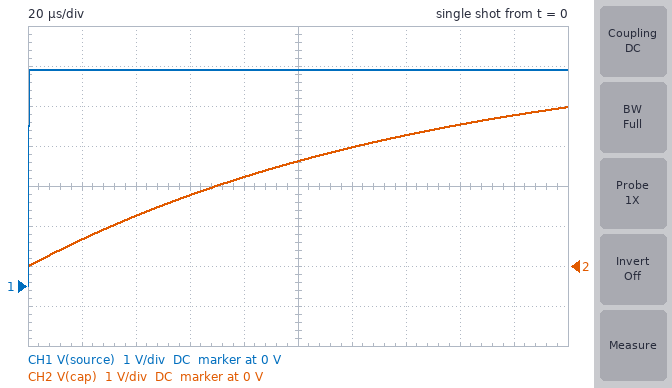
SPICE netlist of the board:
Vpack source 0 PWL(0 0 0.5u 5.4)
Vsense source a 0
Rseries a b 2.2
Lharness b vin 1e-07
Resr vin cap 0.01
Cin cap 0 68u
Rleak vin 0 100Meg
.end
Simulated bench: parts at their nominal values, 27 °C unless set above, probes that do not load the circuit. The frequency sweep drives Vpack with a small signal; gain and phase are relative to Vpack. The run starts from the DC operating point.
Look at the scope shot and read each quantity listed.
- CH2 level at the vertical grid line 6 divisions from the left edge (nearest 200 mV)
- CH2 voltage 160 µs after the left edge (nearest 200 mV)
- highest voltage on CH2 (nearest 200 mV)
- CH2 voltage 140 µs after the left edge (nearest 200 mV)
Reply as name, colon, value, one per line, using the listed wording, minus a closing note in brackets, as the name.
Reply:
CH2 level at the vertical grid line 6 divisions from the left edge: 3.0 V
CH2 voltage 160 µs after the left edge: 3.6 V
highest voltage on CH2: 4.0 V
CH2 voltage 140 µs after the left edge: 3.2 V
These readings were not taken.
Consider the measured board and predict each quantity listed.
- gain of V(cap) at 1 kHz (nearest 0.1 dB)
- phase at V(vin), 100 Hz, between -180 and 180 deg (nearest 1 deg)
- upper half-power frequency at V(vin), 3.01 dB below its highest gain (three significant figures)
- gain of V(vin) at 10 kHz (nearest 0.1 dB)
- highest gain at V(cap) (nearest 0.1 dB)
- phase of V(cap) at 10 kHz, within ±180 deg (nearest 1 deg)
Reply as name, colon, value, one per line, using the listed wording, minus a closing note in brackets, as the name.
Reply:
gain of V(cap) at 1 kHz: -2.8 dB
phase at V(vin), 100 Hz, between -180 and 180 deg: -5 deg
upper half-power frequency at V(vin), 3.01 dB below its highest gain: 1.06 kHz
gain of V(vin) at 10 kHz: -19.5 dB
highest gain at V(cap): 0 dB
phase of V(cap) at 10 kHz, within ±180 deg: -84 deg
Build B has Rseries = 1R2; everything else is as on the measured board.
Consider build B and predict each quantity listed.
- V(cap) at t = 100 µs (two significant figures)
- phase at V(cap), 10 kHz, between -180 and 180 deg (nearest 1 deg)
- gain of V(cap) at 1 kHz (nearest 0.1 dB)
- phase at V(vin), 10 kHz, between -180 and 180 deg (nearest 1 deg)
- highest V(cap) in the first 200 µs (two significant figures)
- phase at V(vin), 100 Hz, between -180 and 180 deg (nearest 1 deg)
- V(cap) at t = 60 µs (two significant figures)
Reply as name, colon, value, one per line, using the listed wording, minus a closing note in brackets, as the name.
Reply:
V(cap) at t = 100 µs: 3.8 V
phase at V(cap), 10 kHz, between -180 and 180 deg: -79 deg
gain of V(cap) at 1 kHz: -1.0 dB
phase at V(vin), 10 kHz, between -180 and 180 deg: -77 deg
highest V(cap) in the first 200 µs: 4.9 V
phase at V(vin), 100 Hz, between -180 and 180 deg: -3 deg
V(cap) at t = 60 µs: 2.8 V
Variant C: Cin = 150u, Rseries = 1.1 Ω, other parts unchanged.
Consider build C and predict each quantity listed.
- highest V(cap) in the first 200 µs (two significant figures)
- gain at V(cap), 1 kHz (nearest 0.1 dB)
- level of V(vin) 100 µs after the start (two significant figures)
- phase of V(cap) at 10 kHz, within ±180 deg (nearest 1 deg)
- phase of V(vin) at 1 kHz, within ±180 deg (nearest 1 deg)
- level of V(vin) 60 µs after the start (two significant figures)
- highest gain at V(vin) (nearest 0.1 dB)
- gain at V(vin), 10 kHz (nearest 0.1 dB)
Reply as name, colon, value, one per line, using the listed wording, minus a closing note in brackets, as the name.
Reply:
highest V(cap) in the first 200 µs: 3.8 V
gain at V(cap), 1 kHz: -3.2 dB
level of V(vin) 100 µs after the start: 2.5 V
phase of V(cap) at 10 kHz, within ±180 deg: -85 deg
phase of V(vin) at 1 kHz, within ±180 deg: -46 deg
level of V(vin) 60 µs after the start: 1.7 V
highest gain at V(vin): 0 dB
gain at V(vin), 10 kHz: -20.4 dB
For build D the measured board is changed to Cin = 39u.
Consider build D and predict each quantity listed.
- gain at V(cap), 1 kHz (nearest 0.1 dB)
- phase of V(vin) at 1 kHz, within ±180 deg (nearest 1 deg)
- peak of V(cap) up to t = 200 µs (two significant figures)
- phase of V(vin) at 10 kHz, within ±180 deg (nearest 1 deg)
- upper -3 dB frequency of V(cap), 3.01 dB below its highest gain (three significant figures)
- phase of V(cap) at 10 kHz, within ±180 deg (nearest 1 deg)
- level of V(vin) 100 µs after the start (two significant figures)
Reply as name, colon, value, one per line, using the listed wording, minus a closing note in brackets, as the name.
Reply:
gain at V(cap), 1 kHz: -1.1 dB
phase of V(vin) at 1 kHz, within ±180 deg: -28 deg
peak of V(cap) up to t = 200 µs: 4.9 V
phase of V(vin) at 10 kHz, within ±180 deg: -78 deg
upper -3 dB frequency of V(cap), 3.01 dB below its highest gain: 1.85 kHz
phase of V(cap) at 10 kHz, within ±180 deg: -80 deg
level of V(vin) 100 µs after the start: 3.7 V
